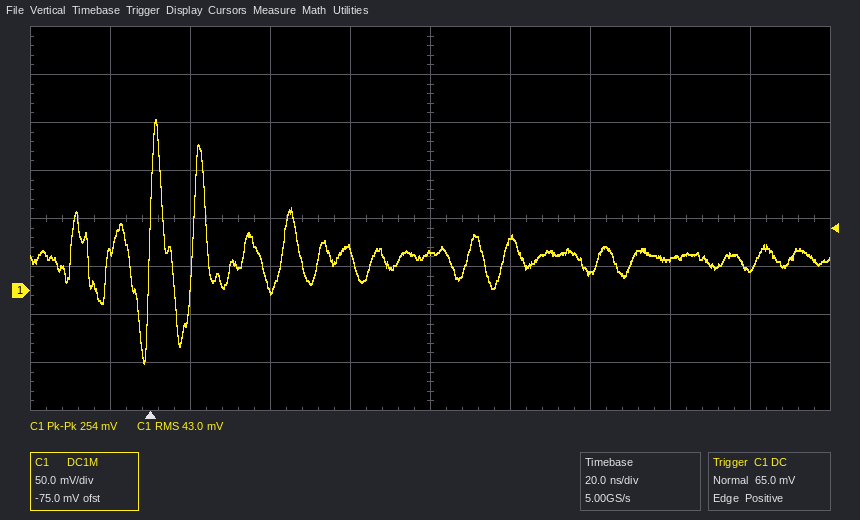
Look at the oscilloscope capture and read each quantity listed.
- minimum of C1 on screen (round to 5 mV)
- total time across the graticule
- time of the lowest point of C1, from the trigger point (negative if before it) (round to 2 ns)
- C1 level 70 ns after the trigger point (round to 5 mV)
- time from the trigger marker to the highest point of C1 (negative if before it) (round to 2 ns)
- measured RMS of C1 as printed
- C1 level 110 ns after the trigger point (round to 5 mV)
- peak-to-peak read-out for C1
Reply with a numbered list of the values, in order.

1. -75 mV
2. 200 ns
3. -2 ns
4. 40 mV
5. +2 ns
6. 43.0 mV
7. 20 mV
8. 254 mV
